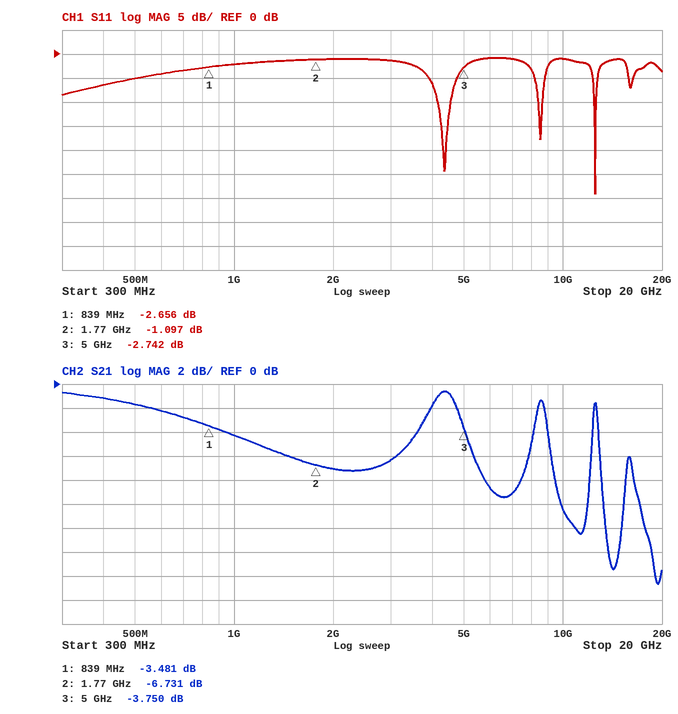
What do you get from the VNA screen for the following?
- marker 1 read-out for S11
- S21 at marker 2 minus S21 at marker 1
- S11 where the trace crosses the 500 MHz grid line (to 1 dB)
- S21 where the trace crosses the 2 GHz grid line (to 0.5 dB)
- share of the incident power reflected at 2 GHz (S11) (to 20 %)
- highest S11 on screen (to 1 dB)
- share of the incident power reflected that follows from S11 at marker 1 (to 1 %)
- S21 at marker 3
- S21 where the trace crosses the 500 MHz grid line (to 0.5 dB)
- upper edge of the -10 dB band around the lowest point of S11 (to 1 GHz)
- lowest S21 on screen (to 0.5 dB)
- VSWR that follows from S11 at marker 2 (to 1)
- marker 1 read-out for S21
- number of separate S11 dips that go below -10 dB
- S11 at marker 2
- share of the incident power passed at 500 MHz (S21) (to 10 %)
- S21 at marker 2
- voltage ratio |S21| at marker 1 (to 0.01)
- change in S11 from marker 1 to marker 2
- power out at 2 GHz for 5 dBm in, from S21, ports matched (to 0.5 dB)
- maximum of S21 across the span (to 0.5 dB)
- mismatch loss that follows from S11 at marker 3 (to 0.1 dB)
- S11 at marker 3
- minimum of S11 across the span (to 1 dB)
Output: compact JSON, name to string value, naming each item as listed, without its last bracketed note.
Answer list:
{"marker 1 read-out for S11": "-2.656 dB", "S21 at marker 2 minus S21 at marker 1": "-3.250 dB", "S11 where the trace crosses the 500 MHz grid line": "-5 dB", "S21 where the trace crosses the 2 GHz grid line": "-7.0 dB", "share of the incident power reflected at 2 GHz (S11)": "80 %", "highest S11 on screen": "-1 dB", "share of the incident power reflected that follows from S11 at marker 1": "54 %", "S21 at marker 3": "-3.750 dB", "S21 where the trace crosses the 500 MHz grid line": "-1.5 dB", "upper edge of the -10 dB band around the lowest point of S11": "13 GHz", "lowest S21 on screen": "-16.5 dB", "VSWR that follows from S11 at marker 2": "16", "marker 1 read-out for S21": "-3.481 dB", "number of separate S11 dips that go below -10 dB": "3", "S11 at marker 2": "-1.097 dB", "share of the incident power passed at 500 MHz (S21)": "70 %", "S21 at marker 2": "-6.731 dB", "voltage ratio |S21| at marker 1": "0.67", "change in S11 from marker 1 to marker 2": "1.559 dB", "power out at 2 GHz for 5 dBm in, from S21, ports matched": "-2.0 dBm", "maximum of S21 across the span": "-0.5 dB", "mismatch loss that follows from S11 at marker 3": "3.3 dB", "S11 at marker 3": "-2.742 dB", "minimum of S11 across the span": "-29 dB"}
